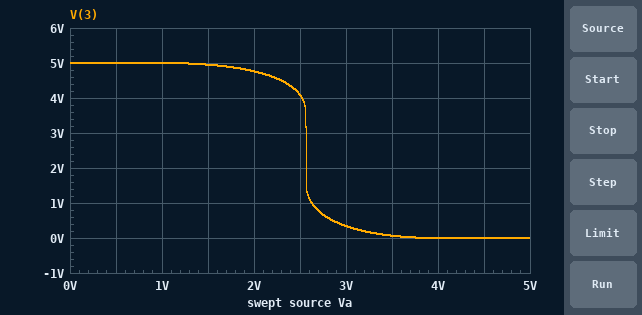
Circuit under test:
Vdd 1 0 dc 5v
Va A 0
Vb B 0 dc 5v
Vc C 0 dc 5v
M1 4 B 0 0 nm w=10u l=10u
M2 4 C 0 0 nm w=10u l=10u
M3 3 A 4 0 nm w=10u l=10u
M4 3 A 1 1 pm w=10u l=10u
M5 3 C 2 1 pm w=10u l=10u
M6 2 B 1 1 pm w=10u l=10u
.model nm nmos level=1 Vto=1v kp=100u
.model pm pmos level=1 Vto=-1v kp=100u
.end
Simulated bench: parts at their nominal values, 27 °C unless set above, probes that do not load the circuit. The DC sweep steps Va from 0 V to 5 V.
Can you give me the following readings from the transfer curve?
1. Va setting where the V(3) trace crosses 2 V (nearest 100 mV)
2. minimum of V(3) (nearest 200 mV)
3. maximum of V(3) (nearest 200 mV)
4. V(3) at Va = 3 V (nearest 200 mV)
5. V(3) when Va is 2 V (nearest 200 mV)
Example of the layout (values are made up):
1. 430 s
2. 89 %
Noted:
1. 2.6 V
2. 0 V
3. 5.0 V
4. 400 mV
5. 4.8 V
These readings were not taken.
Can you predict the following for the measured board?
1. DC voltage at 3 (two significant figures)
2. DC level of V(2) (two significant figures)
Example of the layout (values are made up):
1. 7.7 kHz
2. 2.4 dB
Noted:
1. 5.0 V
2. 5.0 V
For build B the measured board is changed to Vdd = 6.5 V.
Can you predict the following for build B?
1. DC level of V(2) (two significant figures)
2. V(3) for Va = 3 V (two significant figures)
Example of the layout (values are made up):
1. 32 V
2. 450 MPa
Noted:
1. 6.5 V
2. 5.8 V
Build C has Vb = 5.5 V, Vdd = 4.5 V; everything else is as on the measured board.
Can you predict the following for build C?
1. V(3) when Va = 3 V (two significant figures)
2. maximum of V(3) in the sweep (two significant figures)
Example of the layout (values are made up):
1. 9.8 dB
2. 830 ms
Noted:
1. 79 mV
2. 4.5 V
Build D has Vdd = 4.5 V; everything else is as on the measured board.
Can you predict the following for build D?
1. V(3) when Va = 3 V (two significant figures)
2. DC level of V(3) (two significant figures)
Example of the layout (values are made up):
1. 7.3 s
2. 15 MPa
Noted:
1. 80 mV
2. 4.5 V
